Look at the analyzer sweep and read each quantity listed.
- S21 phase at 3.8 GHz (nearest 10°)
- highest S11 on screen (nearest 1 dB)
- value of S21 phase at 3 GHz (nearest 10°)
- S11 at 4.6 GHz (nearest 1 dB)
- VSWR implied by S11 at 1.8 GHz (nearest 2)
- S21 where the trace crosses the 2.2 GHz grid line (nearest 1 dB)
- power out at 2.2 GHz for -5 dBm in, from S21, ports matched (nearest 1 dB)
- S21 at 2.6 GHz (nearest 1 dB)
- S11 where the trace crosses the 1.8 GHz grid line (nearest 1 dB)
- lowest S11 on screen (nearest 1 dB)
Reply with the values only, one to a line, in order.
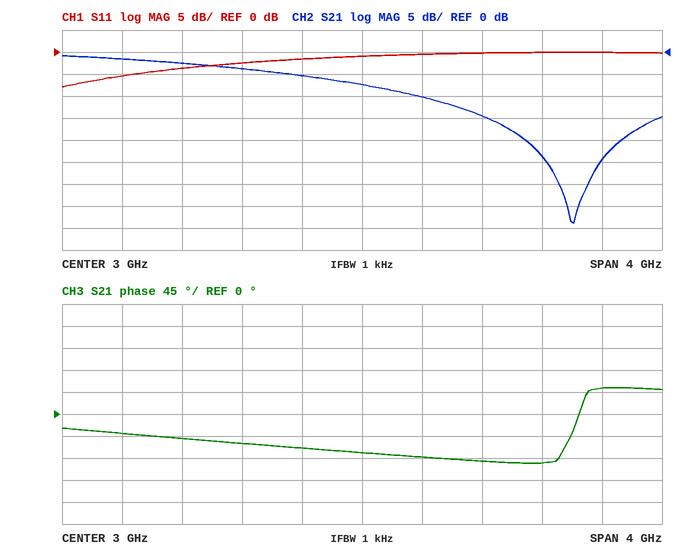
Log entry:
-100°
0 dB
-80°
0 dB
4
-4 dB
-9 dBm
-5 dB
-4 dB
-8 dB
